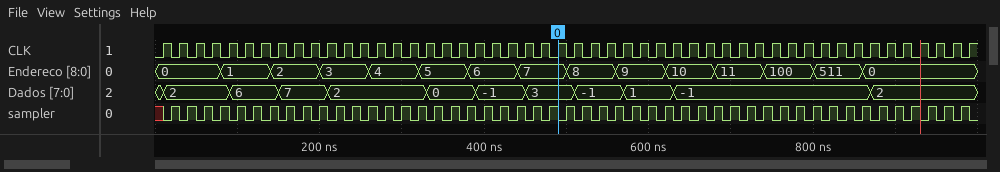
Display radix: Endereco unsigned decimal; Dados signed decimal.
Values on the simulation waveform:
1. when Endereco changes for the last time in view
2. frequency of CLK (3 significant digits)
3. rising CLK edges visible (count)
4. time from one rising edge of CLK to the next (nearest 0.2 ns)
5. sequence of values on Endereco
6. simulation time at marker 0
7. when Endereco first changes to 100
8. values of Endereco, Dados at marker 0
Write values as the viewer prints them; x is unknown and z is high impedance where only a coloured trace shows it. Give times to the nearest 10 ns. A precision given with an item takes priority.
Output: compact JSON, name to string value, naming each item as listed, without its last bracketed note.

{"when Endereco changes for the last time in view": "860 ns", "frequency of CLK": "50.0 MHz", "rising CLK edges visible": "50", "time from one rising edge of CLK to the next": "20 ns", "sequence of values on Endereco": "0, 1, 2, 3, 4, 5, 6, 7, 8, 9, 10, 11, 100, 511, 0", "simulation time at marker 0": "490 ns", "when Endereco first changes to 100": "740 ns", "values of Endereco, Dados at marker 0": "Endereco=7, Dados=3"}
